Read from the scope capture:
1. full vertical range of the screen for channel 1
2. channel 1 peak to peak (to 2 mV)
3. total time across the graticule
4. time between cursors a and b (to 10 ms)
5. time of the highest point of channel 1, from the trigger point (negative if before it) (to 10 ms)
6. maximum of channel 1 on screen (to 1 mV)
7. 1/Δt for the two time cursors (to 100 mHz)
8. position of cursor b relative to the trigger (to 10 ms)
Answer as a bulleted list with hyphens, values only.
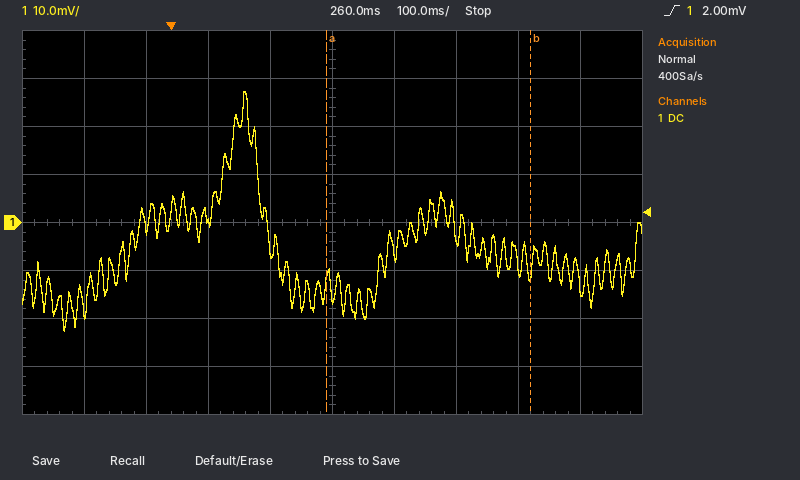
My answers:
- 80 mV
- 50 mV
- 1 s
- 330 ms
- +120 ms
- 27 mV
- 3.0 Hz
- +580 ms
